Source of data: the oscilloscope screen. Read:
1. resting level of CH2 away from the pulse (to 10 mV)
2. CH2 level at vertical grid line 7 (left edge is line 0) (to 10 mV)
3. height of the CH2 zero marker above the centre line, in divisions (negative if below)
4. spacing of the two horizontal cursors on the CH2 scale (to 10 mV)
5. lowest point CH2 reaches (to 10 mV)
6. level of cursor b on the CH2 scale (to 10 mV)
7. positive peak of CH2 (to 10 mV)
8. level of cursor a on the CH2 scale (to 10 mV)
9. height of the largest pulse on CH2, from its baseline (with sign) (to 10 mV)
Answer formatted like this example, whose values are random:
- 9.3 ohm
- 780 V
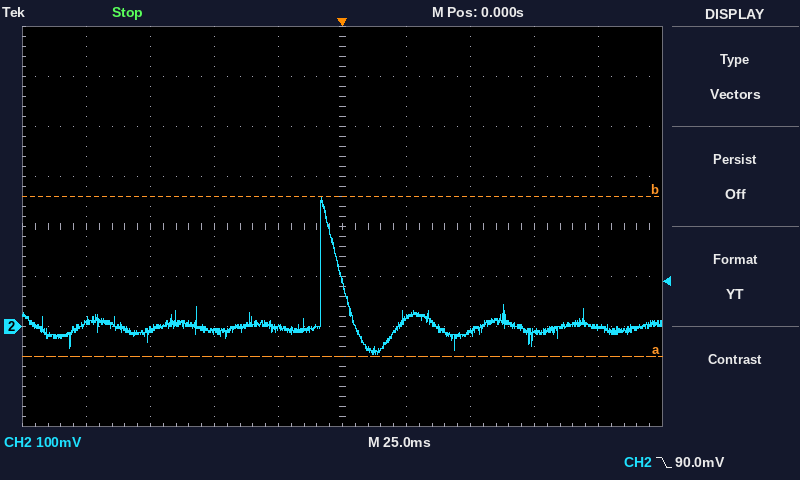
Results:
- 0 mV
- -10 mV
- -2.0 div
- 320 mV
- -60 mV
- 260 mV
- 260 mV
- -60 mV
- +260 mV
